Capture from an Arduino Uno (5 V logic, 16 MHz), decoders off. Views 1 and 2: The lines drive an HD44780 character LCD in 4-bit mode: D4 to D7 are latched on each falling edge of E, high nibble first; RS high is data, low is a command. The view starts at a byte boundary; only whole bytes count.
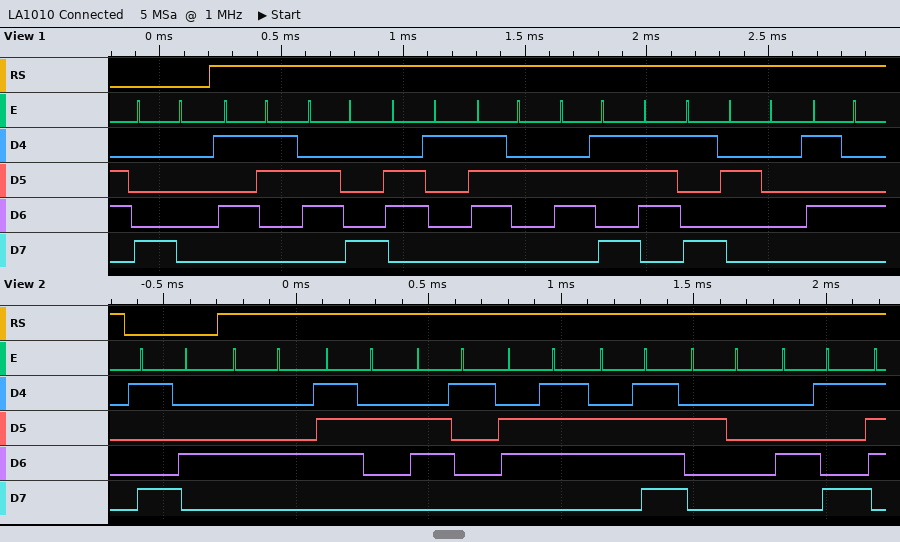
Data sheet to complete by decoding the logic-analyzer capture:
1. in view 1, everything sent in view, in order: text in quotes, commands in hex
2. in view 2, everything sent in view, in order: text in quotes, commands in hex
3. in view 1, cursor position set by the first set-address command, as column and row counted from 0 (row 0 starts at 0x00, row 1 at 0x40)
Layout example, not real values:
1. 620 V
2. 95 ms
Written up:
1. 0x80 "Sharky T"
2. 0x94 "Drago I"
3. column 0, row 0
